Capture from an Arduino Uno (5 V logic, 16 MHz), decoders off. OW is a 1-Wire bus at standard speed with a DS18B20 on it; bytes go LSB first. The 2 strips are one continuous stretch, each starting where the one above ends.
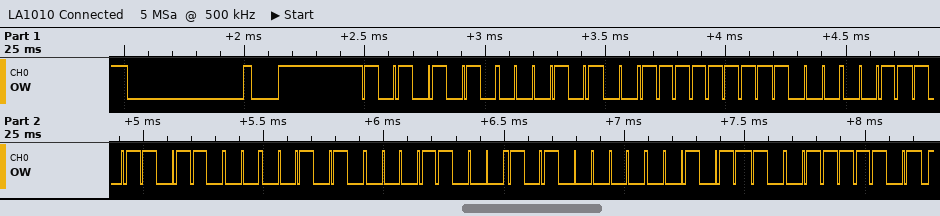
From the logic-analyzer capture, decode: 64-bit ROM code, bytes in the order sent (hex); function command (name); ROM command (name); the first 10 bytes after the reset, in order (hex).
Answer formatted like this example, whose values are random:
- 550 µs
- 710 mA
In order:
- 28 FF C1 6D 50 18 05 74
- Read Scratchpad
- Match ROM
- 55 28 FF C1 6D 50 18 05 74 BE
